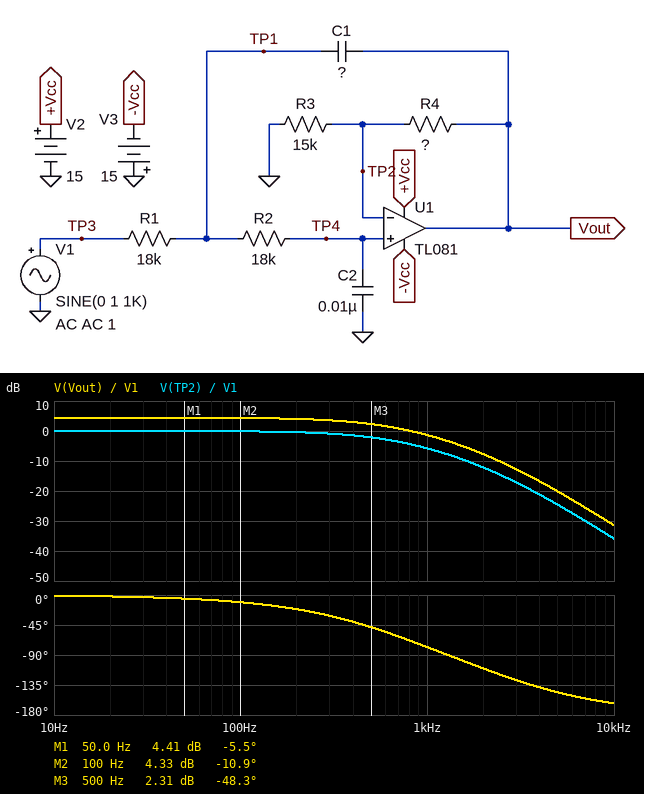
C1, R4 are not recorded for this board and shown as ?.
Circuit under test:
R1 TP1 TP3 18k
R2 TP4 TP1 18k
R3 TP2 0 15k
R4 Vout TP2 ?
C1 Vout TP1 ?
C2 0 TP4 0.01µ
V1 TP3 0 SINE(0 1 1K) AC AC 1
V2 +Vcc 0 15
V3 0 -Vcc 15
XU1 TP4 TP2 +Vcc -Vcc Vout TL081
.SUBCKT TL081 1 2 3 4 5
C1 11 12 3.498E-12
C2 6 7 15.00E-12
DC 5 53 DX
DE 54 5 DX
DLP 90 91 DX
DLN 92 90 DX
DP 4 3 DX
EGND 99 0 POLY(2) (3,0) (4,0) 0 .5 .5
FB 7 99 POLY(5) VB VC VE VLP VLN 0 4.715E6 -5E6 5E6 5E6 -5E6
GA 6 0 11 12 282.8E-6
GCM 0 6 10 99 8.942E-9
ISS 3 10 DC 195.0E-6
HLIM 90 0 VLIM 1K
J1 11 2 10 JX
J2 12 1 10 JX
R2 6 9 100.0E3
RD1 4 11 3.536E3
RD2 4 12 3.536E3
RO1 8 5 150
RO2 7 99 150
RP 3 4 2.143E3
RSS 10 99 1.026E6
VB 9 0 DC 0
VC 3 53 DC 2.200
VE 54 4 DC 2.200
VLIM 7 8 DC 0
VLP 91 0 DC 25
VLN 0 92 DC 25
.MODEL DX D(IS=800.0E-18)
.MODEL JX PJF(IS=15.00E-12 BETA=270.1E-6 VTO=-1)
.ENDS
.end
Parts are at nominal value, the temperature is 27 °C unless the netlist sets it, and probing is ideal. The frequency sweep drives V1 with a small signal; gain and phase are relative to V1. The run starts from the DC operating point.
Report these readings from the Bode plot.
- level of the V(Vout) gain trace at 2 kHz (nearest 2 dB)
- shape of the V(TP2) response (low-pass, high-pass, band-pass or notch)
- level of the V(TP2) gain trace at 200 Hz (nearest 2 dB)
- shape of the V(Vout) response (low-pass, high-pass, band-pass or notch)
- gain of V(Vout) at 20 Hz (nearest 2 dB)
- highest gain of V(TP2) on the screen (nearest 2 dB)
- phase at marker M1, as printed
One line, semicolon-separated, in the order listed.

-8 dB; low-pass; 0 dB; low-pass; 4 dB; 0 dB; -5.5 deg
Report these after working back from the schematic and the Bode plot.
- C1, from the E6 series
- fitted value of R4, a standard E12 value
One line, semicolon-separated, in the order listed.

4.7 nF; 10 kΩ
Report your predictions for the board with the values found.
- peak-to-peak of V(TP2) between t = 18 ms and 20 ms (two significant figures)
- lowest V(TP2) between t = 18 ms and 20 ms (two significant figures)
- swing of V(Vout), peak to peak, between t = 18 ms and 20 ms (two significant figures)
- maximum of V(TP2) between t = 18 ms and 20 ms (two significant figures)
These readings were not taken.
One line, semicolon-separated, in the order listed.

1.0 V; -510 mV; 1.7 V; 510 mV
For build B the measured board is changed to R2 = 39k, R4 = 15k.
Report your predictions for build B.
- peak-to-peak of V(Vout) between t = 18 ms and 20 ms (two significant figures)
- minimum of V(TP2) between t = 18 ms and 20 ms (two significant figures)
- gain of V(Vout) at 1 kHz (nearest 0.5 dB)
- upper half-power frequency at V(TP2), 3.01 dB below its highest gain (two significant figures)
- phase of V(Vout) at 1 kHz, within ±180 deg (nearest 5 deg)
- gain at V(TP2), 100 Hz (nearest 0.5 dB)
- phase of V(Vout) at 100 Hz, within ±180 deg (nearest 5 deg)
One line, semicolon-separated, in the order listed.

1.3 V; -330 mV; -3.5 dB; 380 Hz; -95 deg; -0.5 dB; -15 deg
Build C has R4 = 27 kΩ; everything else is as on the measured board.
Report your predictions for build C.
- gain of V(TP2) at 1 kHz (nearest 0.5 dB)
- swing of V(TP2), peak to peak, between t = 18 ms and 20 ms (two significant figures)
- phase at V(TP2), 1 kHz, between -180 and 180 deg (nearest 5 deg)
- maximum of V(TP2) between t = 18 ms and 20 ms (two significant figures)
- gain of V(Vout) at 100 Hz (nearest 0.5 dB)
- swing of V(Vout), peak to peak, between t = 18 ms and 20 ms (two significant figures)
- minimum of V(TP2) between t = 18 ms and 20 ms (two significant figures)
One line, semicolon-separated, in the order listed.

-2.5 dB; 1.5 V; -75 deg; 730 mV; 9.0 dB; 4.1 V; -730 mV
